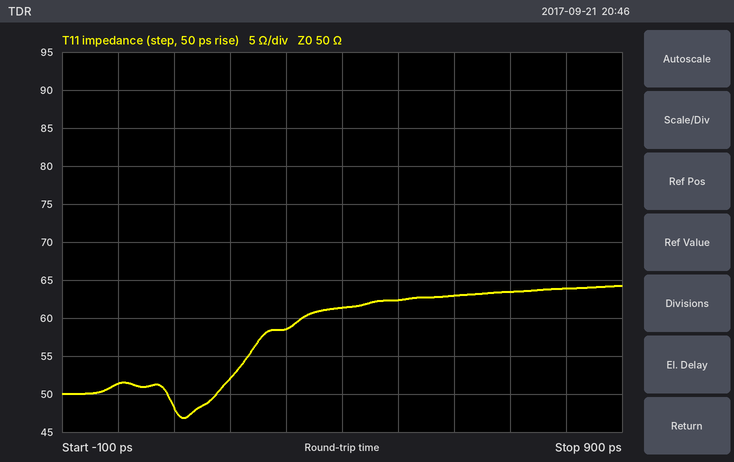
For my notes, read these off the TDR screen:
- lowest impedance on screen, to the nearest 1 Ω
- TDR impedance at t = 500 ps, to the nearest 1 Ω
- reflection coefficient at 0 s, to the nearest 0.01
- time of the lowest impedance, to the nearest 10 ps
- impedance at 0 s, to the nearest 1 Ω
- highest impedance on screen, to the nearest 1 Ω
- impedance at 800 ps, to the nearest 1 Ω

47 Ω
62 Ω
+0.01
120 ps
51 Ω
64 Ω
64 Ω
